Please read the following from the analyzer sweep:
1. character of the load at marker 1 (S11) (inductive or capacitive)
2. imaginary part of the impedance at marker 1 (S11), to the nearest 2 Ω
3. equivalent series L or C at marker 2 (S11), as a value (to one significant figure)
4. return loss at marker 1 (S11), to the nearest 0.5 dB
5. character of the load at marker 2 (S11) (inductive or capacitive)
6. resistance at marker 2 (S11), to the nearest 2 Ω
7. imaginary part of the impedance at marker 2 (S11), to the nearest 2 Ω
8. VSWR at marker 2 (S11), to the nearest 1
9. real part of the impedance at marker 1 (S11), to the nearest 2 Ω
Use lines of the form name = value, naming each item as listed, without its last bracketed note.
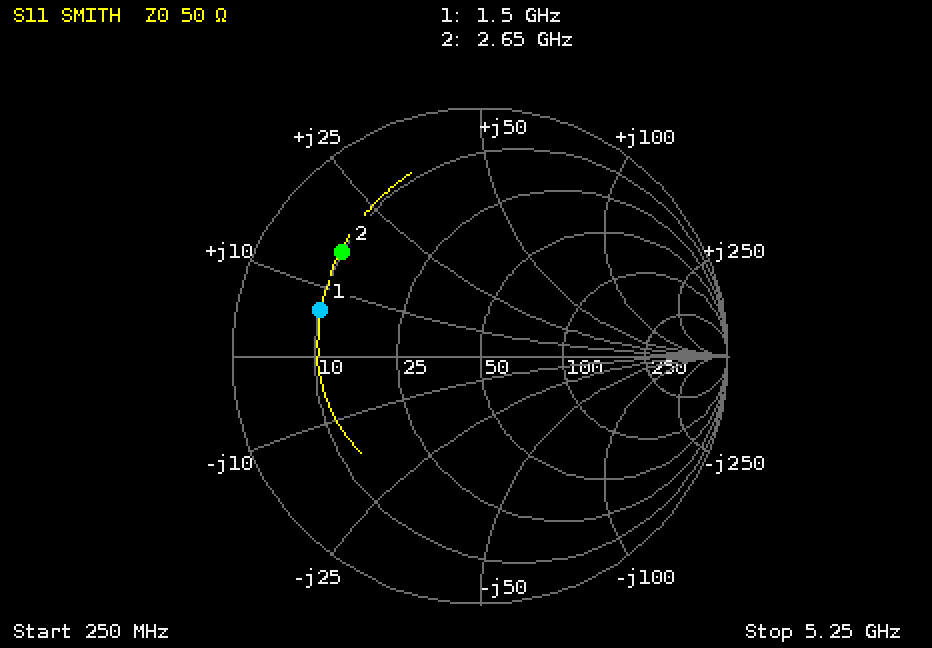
character of the load at marker 1 (S11) = inductive
imaginary part of the impedance at marker 1 (S11), to the nearest 2 Ω = +6 Ω
equivalent series L or C at marker 2 (S11), as a value = 1.0 nH
return loss at marker 1 (S11), to the nearest 0.5 dB = 3.5 dB
character of the load at marker 2 (S11) = inductive
resistance at marker 2 (S11), to the nearest 2 Ω = 10 Ω
imaginary part of the impedance at marker 2 (S11), to the nearest 2 Ω = +16 Ω
VSWR at marker 2 (S11), to the nearest 1 = 6
real part of the impedance at marker 1 (S11), to the nearest 2 Ω = 10 Ω
